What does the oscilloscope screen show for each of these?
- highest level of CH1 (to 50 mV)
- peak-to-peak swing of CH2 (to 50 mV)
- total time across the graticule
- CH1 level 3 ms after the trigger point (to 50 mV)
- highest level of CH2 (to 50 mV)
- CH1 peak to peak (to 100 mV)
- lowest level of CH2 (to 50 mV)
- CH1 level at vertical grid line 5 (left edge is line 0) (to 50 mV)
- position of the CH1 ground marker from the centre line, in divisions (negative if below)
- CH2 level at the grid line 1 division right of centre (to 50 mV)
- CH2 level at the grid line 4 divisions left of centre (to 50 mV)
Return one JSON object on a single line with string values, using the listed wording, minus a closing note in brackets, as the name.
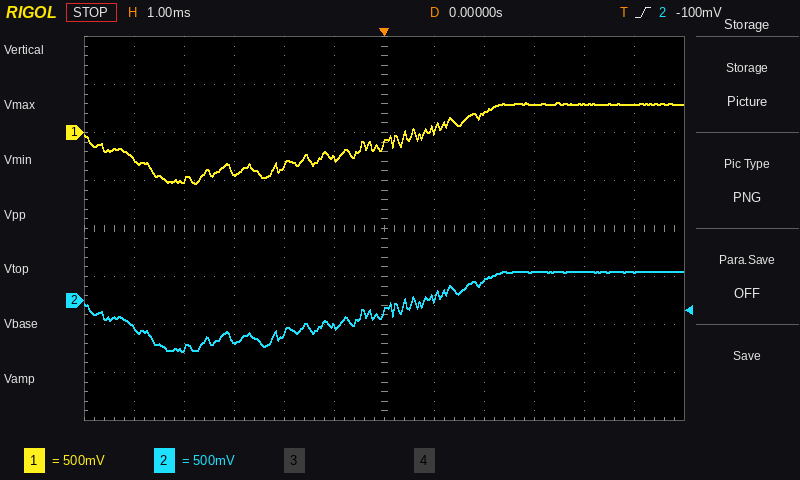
{"highest level of CH1": "300 mV", "peak-to-peak swing of CH2": "850 mV", "total time across the graticule": "12 ms", "CH1 level 3 ms after the trigger point": "300 mV", "highest level of CH2": "300 mV", "CH1 peak to peak": "800 mV", "lowest level of CH2": "-550 mV", "CH1 level at vertical grid line 5 (left edge is line 0)": "-250 mV", "position of the CH1 ground marker from the centre line, in divisions": "+2.0 div", "CH2 level at the grid line 1 division right of centre": "50 mV", "CH2 level at the grid line 4 divisions left of centre": "-500 mV"}
